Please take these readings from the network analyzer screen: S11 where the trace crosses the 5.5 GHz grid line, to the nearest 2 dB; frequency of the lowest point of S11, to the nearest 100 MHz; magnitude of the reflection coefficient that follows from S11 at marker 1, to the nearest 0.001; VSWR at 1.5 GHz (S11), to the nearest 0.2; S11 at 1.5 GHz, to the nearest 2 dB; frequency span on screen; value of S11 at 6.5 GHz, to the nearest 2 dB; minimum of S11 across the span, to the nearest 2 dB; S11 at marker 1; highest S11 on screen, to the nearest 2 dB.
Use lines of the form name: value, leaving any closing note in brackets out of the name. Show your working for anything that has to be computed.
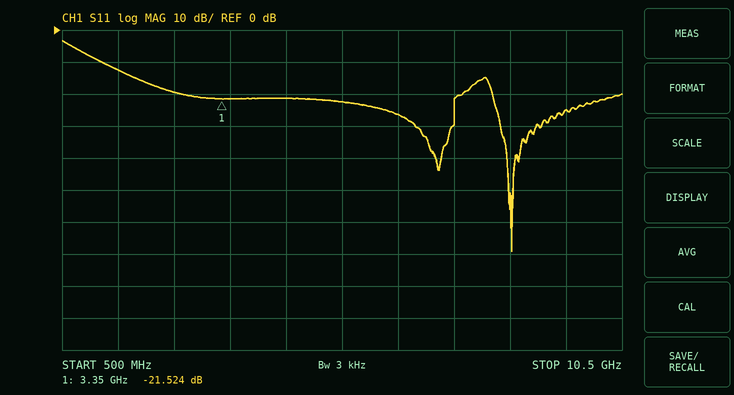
S11 where the trace crosses the 5.5 GHz grid line, to the nearest 2 dB: -22 dB
frequency of the lowest point of S11, to the nearest 100 MHz: 8.5 GHz
magnitude of the reflection coefficient that follows from S11 at marker 1, to the nearest 0.001: 10^(-21.524/20) ≈ 0.084
VSWR at 1.5 GHz (S11), to the nearest 0.2: |Γ| = 10^(-12/20) = 0.2512; VSWR = (1 + 0.2512)/(1 − 0.2512) ≈ 1.67, so 1.6 to the nearest 0.2
S11 at 1.5 GHz, to the nearest 2 dB: -12 dB
frequency span on screen: 10 GHz
value of S11 at 6.5 GHz, to the nearest 2 dB: -26 dB
minimum of S11 across the span, to the nearest 2 dB: -70 dB
S11 at marker 1: -21.524 dB
highest S11 on screen, to the nearest 2 dB: -4 dB
